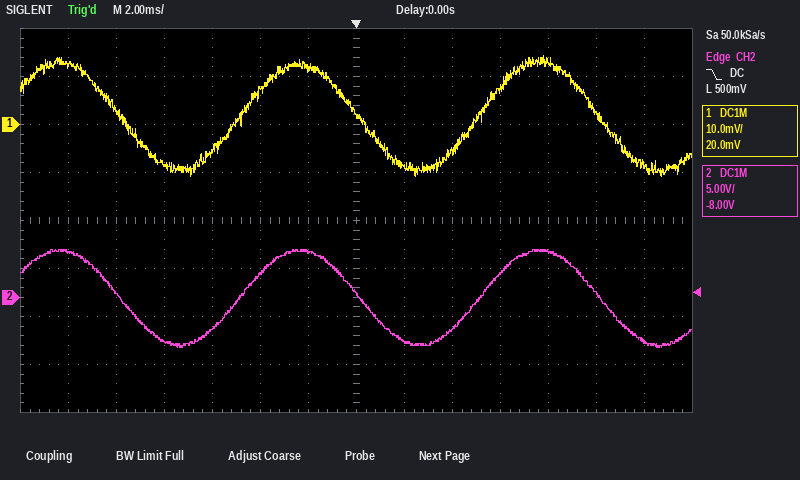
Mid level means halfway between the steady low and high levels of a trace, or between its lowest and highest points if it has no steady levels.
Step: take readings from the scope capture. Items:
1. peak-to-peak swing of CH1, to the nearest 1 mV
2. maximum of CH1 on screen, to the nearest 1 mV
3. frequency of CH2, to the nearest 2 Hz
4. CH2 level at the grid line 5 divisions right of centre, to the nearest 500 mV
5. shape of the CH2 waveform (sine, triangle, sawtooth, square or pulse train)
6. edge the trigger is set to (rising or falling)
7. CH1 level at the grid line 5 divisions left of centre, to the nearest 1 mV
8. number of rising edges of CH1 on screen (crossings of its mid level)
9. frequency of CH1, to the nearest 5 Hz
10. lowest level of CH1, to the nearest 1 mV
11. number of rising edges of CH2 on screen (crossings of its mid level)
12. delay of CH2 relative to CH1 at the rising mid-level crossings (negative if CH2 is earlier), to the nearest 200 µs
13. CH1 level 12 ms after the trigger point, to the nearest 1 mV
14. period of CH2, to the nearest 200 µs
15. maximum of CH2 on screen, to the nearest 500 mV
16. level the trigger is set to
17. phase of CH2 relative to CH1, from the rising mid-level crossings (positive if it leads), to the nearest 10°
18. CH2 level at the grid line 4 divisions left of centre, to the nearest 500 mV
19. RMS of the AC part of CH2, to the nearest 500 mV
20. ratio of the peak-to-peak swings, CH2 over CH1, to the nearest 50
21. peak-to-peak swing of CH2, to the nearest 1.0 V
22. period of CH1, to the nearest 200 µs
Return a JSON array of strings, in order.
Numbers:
["25 mV", "14 mV", "100 Hz", "500 mV", "sine", "falling", "3 mV", "2", "100 Hz", "-11 mV", "2", "0.0 ms", "-8 mV", "10.0 ms", "5.0 V", "500 mV", "0°", "-4.5 V", "3.5 V", "400", "10.0 V", "10.0 ms"]
